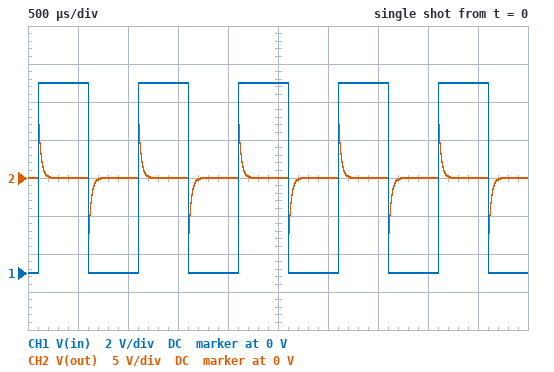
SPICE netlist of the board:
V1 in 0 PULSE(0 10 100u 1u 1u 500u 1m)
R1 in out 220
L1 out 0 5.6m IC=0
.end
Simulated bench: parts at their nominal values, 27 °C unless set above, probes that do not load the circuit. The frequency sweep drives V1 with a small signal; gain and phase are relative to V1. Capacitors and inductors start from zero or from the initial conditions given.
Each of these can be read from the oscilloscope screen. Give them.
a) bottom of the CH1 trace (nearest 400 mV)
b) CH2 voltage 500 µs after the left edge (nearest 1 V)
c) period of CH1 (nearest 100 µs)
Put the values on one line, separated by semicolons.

0 V; 0 V; 1.0 ms
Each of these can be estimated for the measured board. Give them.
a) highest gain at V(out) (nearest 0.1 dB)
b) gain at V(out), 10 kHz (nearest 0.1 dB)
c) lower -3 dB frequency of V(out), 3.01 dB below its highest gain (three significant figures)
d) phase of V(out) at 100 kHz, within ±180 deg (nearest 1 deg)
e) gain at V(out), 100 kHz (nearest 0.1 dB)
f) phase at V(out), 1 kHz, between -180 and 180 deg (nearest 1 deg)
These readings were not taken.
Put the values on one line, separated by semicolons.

0 dB; -1.4 dB; 6.25 kHz; 4 deg; 0 dB; 81 deg
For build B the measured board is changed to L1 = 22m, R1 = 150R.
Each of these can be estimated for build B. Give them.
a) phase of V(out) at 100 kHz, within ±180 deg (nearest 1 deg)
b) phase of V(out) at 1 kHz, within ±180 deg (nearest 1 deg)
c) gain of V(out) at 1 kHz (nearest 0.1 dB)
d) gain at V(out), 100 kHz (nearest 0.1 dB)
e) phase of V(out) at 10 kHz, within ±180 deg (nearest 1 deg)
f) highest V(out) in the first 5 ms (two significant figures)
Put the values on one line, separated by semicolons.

1 deg; 47 deg; -3.4 dB; 0 dB; 6 deg; 10 V
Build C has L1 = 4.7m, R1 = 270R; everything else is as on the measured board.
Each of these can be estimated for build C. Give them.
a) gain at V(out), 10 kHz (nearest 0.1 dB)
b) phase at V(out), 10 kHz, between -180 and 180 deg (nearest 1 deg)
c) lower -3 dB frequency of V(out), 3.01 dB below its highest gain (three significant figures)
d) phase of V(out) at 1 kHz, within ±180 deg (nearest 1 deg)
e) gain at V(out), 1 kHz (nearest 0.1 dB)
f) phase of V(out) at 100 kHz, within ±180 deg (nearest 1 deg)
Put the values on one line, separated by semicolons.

-2.6 dB; 42 deg; 9.14 kHz; 84 deg; -19.3 dB; 5 deg
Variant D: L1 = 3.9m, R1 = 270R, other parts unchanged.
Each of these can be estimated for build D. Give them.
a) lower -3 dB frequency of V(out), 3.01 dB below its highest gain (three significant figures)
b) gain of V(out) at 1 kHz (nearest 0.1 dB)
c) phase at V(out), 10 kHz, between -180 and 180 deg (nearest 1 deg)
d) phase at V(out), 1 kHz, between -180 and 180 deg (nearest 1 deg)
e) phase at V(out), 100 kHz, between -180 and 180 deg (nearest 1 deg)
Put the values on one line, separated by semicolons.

11.0 kHz; -20.9 dB; 48 deg; 85 deg; 6 deg
